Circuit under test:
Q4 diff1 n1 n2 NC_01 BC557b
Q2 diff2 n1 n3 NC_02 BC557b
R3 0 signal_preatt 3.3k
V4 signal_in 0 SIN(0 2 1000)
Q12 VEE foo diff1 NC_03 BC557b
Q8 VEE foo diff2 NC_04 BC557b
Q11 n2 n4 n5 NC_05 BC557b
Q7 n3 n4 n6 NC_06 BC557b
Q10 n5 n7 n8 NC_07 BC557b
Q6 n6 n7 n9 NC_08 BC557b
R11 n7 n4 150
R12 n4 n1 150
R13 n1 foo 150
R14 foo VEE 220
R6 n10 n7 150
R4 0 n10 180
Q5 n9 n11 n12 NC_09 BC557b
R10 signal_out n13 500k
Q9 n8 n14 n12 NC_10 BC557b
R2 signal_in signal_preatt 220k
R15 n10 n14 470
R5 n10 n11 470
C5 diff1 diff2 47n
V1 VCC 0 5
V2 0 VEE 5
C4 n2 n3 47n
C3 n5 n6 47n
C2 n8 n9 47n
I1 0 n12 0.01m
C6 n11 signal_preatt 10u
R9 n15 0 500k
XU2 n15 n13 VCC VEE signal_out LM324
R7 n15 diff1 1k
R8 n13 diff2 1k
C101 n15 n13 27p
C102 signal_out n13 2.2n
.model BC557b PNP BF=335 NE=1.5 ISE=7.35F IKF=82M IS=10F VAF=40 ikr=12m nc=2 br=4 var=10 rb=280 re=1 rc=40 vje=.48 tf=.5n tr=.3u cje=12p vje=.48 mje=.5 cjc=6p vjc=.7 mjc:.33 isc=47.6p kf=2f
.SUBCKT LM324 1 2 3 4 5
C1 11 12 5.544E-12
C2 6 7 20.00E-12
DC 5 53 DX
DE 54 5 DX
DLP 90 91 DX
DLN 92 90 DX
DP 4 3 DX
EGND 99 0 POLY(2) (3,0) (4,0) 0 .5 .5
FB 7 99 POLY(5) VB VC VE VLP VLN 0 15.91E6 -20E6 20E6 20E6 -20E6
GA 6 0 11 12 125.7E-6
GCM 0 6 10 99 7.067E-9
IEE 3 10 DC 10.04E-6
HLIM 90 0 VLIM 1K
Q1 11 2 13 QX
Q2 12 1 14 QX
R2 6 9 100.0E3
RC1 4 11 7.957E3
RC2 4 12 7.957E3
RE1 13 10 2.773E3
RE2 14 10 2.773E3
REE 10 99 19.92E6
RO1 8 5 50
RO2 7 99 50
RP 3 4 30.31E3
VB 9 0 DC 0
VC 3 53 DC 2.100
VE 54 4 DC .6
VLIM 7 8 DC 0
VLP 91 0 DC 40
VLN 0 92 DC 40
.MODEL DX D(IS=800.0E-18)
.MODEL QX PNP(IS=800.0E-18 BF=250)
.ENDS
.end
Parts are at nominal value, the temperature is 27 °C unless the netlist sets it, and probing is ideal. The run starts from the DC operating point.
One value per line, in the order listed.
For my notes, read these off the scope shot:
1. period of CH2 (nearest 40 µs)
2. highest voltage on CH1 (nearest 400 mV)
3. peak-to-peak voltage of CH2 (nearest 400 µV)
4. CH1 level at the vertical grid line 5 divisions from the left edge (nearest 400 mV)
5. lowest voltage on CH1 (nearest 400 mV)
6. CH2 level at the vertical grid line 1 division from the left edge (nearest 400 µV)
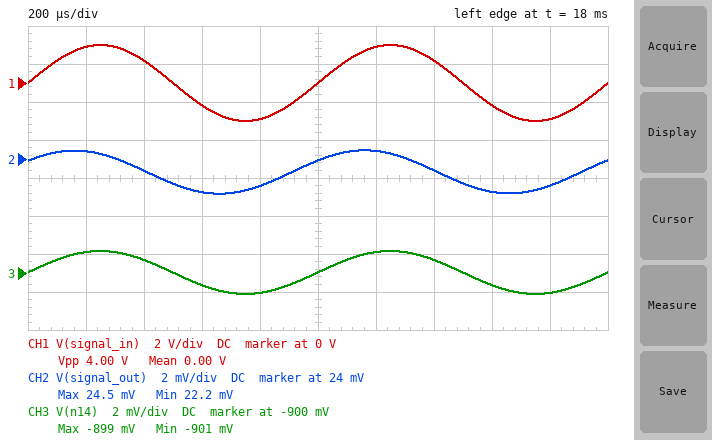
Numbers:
1.00 ms
2.0 V
2.4 mV
0 V
-2.0 V
24.4 mV
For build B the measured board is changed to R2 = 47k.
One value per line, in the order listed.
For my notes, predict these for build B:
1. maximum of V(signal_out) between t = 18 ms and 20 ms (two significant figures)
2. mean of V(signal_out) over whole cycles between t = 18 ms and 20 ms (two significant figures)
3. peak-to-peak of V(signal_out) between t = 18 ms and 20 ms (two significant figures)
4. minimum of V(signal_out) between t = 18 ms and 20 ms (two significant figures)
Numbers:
26 mV
21 mV
10 mV
16 mV
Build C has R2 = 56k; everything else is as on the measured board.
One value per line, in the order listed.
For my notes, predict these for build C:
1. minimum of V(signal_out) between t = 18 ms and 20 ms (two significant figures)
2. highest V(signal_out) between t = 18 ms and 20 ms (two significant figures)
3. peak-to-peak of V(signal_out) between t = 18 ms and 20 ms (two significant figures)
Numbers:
17 mV
26 mV
8.8 mV
